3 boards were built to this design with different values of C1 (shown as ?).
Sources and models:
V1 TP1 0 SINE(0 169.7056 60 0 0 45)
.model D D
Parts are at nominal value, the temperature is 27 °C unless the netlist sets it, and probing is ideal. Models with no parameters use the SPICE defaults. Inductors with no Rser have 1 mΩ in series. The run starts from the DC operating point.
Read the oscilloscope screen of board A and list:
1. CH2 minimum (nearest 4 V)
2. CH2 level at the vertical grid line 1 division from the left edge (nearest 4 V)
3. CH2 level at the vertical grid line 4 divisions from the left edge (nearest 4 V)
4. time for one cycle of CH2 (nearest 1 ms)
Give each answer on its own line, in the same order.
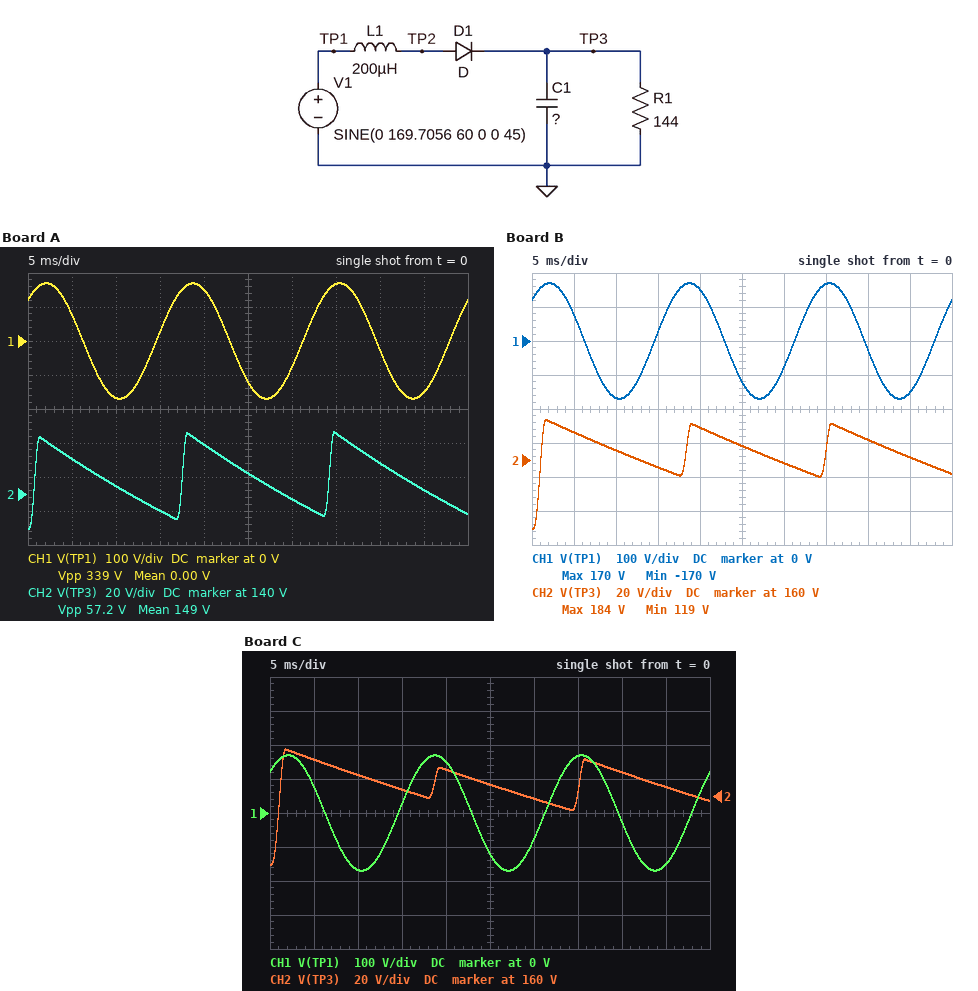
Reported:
120 V
160 V
168 V
17 ms
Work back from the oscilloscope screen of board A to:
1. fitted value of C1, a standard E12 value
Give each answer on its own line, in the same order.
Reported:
330 µF
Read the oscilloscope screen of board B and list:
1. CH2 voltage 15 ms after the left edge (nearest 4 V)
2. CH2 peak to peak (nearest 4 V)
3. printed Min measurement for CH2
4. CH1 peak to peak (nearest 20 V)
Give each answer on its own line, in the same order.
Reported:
156 V
64 V
119 V
340 V
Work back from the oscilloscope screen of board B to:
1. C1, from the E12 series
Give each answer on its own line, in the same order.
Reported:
560 µF
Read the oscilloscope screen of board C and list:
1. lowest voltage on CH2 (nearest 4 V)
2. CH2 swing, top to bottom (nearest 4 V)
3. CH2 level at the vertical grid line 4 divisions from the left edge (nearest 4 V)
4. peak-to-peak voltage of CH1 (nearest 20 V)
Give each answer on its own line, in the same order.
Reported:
120 V
68 V
176 V
340 V
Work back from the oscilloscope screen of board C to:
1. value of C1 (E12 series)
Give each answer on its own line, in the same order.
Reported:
680 µF
